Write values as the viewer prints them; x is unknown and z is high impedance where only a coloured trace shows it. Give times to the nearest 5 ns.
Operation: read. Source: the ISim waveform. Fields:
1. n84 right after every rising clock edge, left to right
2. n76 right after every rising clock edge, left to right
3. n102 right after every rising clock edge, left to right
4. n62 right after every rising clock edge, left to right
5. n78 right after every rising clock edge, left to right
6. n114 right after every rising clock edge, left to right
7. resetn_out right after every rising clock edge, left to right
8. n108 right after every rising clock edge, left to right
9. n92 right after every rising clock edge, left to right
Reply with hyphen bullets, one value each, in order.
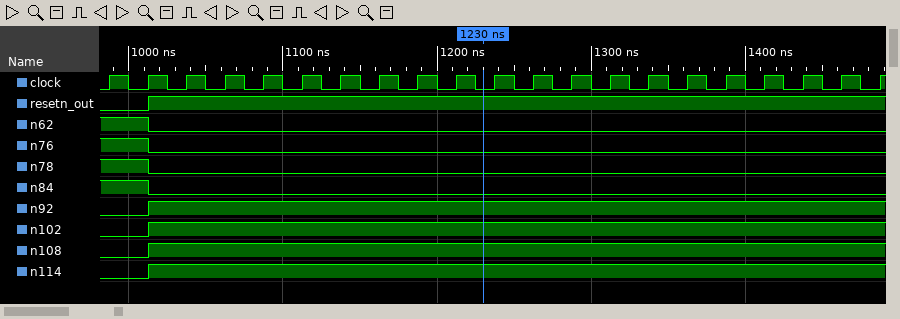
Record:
- 1 0 0 0 0 0 0 0 0 0 0 0 0 0 0 0 0 0 0 0 0
- 1 0 0 0 0 0 0 0 0 0 0 0 0 0 0 0 0 0 0 0 0
- 0 1 1 1 1 1 1 1 1 1 1 1 1 1 1 1 1 1 1 1 1
- 1 0 0 0 0 0 0 0 0 0 0 0 0 0 0 0 0 0 0 0 0
- 1 0 0 0 0 0 0 0 0 0 0 0 0 0 0 0 0 0 0 0 0
- 0 1 1 1 1 1 1 1 1 1 1 1 1 1 1 1 1 1 1 1 1
- 0 1 1 1 1 1 1 1 1 1 1 1 1 1 1 1 1 1 1 1 1
- 0 1 1 1 1 1 1 1 1 1 1 1 1 1 1 1 1 1 1 1 1
- 0 1 1 1 1 1 1 1 1 1 1 1 1 1 1 1 1 1 1 1 1
